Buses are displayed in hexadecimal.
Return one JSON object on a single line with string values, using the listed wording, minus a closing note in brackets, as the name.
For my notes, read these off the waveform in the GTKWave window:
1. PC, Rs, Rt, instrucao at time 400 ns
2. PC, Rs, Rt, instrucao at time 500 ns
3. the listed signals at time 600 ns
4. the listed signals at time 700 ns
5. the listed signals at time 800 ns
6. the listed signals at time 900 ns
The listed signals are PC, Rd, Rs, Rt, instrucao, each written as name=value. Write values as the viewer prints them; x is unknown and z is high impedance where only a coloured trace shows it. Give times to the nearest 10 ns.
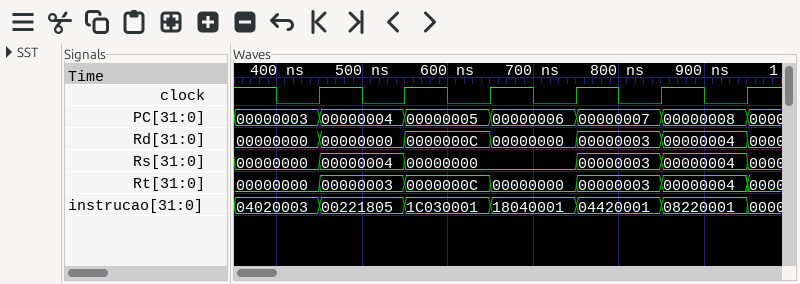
{"PC, Rs, Rt, instrucao at time 400 ns": "PC=00000003, Rs=00000000, Rt=00000000, instrucao=04020003", "PC, Rs, Rt, instrucao at time 500 ns": "PC=00000004, Rs=00000004, Rt=00000003, instrucao=00221805", "the listed signals at time 600 ns": "PC=00000005, Rd=0000000C, Rs=00000000, Rt=0000000C, instrucao=1C030001", "the listed signals at time 700 ns": "PC=00000006, Rd=00000000, Rs=00000000, Rt=00000000, instrucao=18040001", "the listed signals at time 800 ns": "PC=00000007, Rd=00000003, Rs=00000003, Rt=00000003, instrucao=04420001", "the listed signals at time 900 ns": "PC=00000008, Rd=00000004, Rs=00000004, Rt=00000004, instrucao=08220001"}
